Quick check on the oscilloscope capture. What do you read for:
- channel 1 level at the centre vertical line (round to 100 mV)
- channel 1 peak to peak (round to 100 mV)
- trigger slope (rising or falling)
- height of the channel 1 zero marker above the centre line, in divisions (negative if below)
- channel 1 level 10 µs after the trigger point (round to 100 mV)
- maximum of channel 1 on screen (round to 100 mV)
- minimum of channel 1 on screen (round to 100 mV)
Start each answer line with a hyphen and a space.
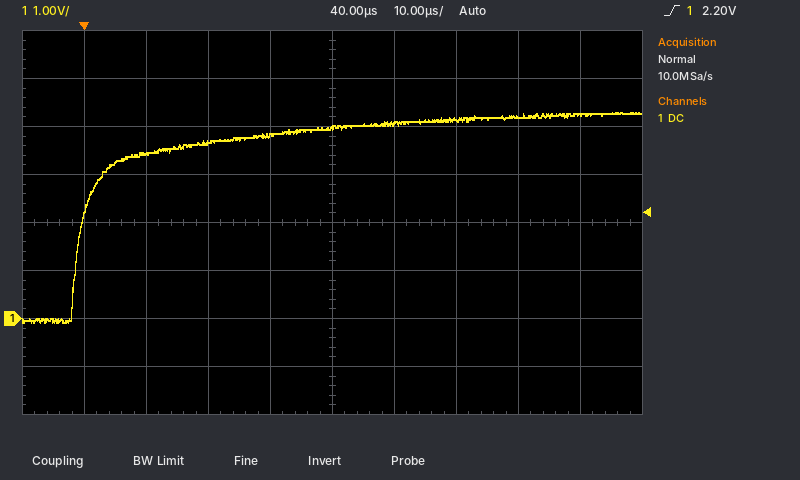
- 4.0 V
- 4.4 V
- rising
- -2.0 div
- 3.4 V
- 4.3 V
- -100 mV
